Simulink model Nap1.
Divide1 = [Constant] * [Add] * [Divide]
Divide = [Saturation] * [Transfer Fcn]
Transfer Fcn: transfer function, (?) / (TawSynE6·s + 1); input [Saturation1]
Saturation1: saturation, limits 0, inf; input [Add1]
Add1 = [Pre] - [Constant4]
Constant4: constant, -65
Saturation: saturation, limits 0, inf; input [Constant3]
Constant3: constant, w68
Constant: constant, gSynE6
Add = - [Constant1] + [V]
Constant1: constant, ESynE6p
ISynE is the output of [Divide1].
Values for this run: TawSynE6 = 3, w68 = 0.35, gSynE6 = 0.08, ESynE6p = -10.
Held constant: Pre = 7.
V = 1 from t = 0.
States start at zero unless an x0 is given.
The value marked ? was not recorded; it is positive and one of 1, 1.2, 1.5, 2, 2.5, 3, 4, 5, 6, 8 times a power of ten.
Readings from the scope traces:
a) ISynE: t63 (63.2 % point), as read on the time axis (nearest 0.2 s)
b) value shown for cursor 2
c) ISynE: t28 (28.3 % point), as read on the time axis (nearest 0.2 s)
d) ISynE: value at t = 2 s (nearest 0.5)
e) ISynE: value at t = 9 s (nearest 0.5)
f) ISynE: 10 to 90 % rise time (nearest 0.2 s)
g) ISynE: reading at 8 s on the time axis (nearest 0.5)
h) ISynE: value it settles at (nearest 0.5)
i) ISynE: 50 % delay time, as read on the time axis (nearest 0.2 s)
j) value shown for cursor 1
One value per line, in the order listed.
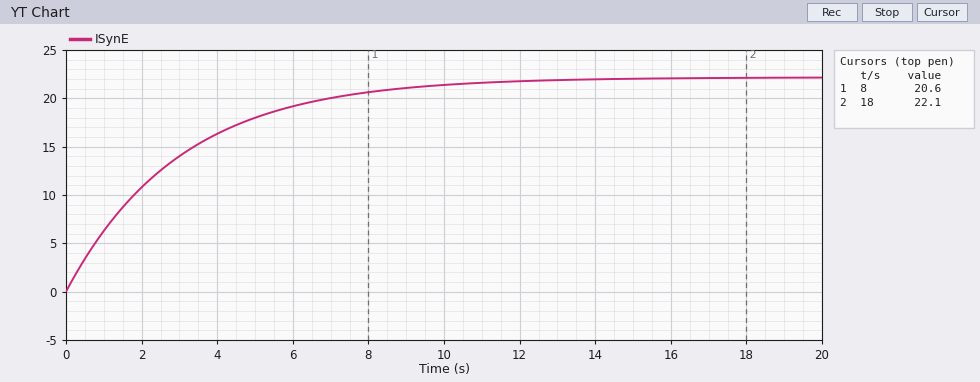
3.0 s
22.1
1.0 s
11.0
21.0
6.6 s
20.5
22.0
2.0 s
20.6
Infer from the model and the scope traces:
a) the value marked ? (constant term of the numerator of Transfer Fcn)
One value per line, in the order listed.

1
